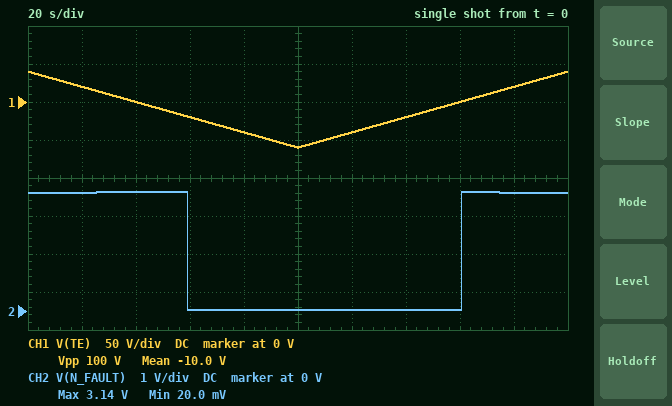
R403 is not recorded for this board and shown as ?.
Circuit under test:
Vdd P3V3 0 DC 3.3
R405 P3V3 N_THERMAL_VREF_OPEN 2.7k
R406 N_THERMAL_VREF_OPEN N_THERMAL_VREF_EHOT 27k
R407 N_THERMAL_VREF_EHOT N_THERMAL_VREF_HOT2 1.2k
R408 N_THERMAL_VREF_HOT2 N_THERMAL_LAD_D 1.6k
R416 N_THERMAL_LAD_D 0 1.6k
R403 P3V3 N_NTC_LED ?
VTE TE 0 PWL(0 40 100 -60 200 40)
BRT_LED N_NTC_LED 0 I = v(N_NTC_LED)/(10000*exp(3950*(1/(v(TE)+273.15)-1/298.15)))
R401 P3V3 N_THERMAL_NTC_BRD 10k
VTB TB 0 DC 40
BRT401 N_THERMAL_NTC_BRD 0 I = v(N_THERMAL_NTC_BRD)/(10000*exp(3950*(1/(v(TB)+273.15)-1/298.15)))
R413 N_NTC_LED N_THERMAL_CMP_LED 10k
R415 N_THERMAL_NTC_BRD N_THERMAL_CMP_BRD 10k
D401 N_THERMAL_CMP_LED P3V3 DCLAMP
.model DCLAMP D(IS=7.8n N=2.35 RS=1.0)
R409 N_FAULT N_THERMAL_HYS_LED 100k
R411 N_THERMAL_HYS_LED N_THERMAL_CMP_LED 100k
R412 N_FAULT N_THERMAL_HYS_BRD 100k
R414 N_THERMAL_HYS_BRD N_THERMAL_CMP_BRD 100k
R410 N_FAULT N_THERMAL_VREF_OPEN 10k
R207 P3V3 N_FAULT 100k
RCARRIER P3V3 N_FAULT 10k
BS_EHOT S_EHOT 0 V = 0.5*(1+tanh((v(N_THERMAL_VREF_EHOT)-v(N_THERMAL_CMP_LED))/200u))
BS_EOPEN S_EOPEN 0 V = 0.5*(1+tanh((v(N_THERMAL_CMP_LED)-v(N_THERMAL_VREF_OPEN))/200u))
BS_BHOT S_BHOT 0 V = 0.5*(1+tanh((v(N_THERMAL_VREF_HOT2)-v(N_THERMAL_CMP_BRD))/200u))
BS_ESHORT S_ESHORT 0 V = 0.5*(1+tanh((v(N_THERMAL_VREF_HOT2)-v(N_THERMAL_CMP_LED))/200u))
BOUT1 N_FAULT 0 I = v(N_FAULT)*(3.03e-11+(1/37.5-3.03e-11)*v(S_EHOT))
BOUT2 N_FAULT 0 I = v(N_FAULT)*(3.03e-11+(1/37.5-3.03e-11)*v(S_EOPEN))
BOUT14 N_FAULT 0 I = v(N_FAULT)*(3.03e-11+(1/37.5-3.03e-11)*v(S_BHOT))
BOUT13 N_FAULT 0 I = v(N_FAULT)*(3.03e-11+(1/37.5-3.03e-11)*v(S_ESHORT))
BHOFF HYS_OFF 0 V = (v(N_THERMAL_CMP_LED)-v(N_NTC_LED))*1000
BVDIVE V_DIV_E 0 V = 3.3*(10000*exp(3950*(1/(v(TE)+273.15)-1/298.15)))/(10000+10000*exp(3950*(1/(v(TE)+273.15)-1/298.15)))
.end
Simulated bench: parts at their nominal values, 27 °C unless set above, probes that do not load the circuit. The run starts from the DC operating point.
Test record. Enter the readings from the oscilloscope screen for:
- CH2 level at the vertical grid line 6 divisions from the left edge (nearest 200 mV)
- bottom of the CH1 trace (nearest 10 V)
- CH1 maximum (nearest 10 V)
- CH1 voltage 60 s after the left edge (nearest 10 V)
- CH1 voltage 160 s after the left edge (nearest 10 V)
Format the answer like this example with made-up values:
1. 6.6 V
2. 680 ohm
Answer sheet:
1. 0 V
2. -60 V
3. 40 V
4. -20 V
5. 0 V
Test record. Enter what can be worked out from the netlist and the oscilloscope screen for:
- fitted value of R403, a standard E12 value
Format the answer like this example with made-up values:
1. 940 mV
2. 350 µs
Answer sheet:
1. 8.2 kΩ
